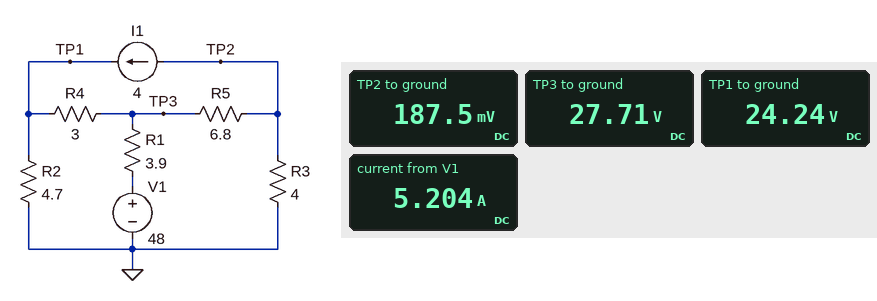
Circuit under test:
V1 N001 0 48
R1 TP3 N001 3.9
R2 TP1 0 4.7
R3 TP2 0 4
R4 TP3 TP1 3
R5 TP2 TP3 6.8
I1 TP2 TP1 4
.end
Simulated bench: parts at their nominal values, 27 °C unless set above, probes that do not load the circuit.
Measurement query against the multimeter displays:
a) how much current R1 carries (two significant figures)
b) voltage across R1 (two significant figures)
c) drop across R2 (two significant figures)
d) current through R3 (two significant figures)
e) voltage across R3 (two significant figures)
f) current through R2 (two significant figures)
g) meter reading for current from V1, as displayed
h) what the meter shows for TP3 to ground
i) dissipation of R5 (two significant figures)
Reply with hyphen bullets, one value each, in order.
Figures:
- 5.2 A
- 20 V
- 24 V
- 47 mA
- 190 mV
- 5.2 A
- 5.204 A
- 27.71 V
- 110 W
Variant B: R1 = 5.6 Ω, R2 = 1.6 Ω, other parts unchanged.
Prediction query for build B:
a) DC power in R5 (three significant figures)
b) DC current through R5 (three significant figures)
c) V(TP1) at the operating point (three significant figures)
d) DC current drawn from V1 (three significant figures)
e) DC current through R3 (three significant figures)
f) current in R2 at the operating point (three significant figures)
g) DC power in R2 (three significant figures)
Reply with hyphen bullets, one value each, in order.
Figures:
- 64.9 W
- 3.09 A
- 10.2 V
- 5.47 A
- 911 mA
- 6.38 A
- 65.2 W
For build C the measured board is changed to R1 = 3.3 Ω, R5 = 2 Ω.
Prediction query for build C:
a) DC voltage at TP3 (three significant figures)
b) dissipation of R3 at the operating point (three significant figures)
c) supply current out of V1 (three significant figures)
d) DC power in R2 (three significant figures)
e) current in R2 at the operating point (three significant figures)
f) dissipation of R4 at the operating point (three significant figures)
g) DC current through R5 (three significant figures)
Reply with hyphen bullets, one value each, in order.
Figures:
- 23.9 V
- 28.0 W
- 7.31 A
- 102 W
- 4.66 A
- 1.31 W
- 6.65 A
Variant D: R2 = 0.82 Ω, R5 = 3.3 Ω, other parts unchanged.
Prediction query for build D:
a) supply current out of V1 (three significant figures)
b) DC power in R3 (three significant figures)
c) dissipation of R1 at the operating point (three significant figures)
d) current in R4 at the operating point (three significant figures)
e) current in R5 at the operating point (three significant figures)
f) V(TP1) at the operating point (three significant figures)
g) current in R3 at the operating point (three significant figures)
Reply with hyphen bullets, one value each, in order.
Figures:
- 8.01 A
- 946 mW
- 250 W
- 3.53 A
- 4.49 A
- 6.17 V
- 486 mA
